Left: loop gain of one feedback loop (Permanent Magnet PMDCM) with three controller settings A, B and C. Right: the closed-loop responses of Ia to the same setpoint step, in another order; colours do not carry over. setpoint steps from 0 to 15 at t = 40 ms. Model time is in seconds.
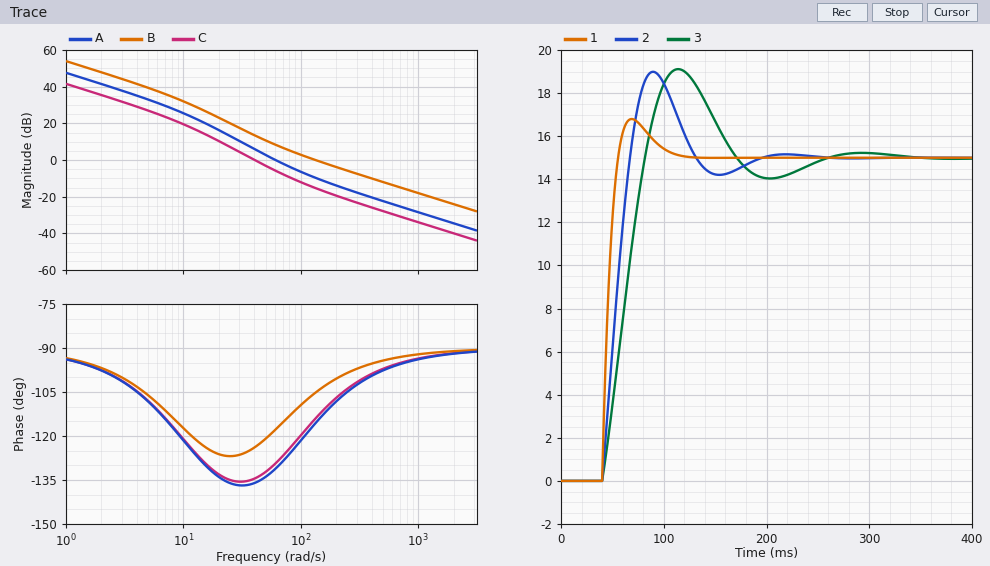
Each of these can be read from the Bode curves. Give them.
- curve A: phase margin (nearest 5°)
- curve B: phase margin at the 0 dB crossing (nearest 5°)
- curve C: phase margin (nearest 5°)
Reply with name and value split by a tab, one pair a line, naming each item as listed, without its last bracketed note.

curve A: phase margin	50°
curve B: phase margin at the 0 dB crossing	75°
curve C: phase margin	45°
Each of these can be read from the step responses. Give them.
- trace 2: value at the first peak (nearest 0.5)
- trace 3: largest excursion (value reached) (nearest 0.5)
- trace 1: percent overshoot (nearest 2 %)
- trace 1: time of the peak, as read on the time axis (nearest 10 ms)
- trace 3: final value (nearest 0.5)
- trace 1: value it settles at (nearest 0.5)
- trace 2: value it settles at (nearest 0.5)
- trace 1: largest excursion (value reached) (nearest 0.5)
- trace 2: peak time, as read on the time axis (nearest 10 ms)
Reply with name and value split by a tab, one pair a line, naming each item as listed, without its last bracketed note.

trace 2: value at the first peak	19.0
trace 3: largest excursion (value reached)	19.0
trace 1: percent overshoot	12 %
trace 1: time of the peak, as read on the time axis	70 ms
trace 3: final value	15.0
trace 1: value it settles at	15.0
trace 2: value it settles at	15.0
trace 1: largest excursion (value reached)	17.0
trace 2: peak time, as read on the time axis	90 ms
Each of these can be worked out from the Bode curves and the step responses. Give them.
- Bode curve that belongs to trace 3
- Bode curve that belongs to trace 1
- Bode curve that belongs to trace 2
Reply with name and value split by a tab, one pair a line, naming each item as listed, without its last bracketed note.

Bode curve that belongs to trace 3	C
Bode curve that belongs to trace 1	B
Bode curve that belongs to trace 2	A
